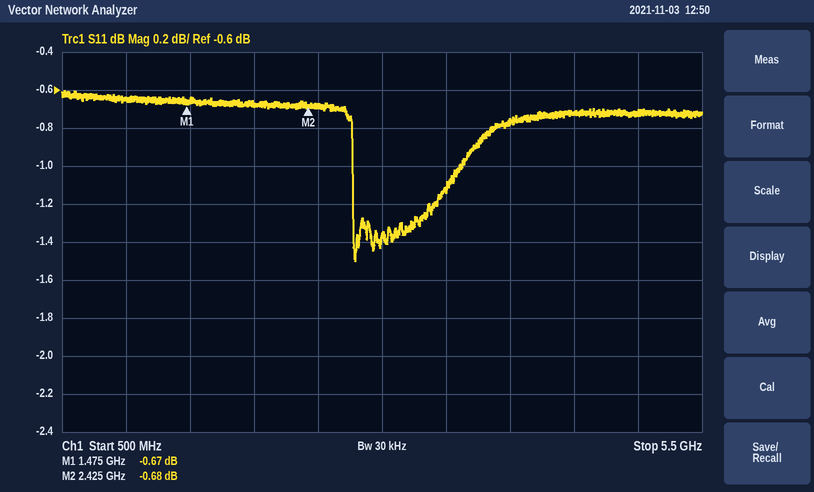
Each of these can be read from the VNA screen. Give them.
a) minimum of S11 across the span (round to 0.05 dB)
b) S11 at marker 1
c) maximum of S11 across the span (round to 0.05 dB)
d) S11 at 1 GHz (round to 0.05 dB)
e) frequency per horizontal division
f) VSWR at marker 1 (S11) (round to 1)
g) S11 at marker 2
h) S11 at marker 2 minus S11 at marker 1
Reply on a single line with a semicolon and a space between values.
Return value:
-1.50 dB; -0.67 dB; -0.60 dB; -0.65 dB; 500 MHz; 26; -0.68 dB; -0.01 dB
